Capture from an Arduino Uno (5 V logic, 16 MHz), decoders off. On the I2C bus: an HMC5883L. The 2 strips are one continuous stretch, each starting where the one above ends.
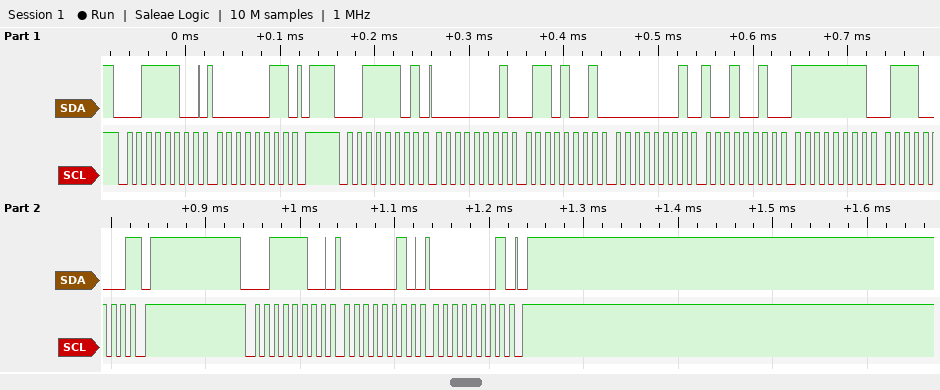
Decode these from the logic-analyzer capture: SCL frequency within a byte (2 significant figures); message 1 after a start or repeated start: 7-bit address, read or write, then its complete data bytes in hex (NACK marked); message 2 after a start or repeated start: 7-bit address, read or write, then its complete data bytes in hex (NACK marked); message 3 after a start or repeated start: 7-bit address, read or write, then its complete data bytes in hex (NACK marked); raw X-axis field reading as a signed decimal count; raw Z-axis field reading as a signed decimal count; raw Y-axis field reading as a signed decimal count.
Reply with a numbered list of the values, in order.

1. 100 kHz
2. 0x1E write: 03
3. 0x1E read: 01 69 01 92 FF 70 NACK
4. 0x1E write: 02 01
5. 361
6. 402
7. -144
